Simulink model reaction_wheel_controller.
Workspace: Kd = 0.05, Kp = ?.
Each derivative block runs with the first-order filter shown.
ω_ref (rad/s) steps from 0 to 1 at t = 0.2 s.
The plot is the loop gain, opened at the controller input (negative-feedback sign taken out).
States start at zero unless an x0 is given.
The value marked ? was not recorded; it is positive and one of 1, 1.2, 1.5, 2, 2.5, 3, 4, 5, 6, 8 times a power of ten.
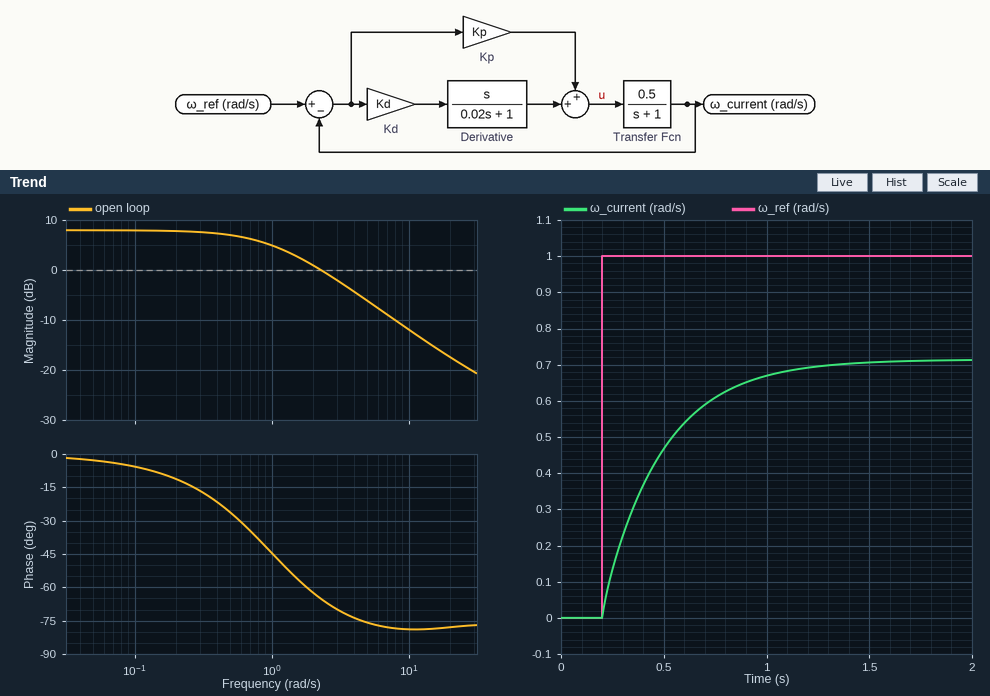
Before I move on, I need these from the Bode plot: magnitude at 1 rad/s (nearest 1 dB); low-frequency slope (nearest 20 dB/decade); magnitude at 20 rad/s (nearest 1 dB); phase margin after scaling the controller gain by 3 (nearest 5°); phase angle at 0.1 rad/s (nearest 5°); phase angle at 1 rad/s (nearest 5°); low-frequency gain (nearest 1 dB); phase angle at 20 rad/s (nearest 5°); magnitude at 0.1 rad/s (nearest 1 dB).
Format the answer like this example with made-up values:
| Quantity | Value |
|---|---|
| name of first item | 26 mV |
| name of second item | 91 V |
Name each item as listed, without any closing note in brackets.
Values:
| Quantity | Value |
|---|---|
| magnitude at 1 rad/s | 5 dB |
| low-frequency slope | 0 dB/decade |
| magnitude at 20 rad/s | -17 dB |
| phase margin after scaling the controller gain by 3 | 100° |
| phase angle at 0.1 rad/s | -5° |
| phase angle at 1 rad/s | -45° |
| low-frequency gain | 8 dB |
| phase angle at 20 rad/s | -80° |
| magnitude at 0.1 rad/s | 8 dB |
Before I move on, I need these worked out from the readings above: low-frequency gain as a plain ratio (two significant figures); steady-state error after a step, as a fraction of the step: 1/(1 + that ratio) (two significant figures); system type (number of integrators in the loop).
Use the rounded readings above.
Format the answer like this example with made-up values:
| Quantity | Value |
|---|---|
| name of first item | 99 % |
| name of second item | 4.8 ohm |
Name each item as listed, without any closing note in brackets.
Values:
| Quantity | Value |
|---|---|
| low-frequency gain as a plain ratio | 2.5 |
| steady-state error after a step, as a fraction of the step: 1/(1 + that ratio) | 0.29 |
| system type | 0 |
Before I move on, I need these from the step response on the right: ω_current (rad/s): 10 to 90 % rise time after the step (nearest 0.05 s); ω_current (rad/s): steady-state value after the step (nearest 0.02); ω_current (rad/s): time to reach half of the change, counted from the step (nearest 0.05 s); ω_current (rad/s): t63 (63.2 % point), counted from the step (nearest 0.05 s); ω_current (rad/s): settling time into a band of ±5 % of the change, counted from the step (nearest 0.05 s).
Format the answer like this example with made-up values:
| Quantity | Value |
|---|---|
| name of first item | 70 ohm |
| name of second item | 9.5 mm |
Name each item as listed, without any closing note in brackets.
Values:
| Quantity | Value |
|---|---|
| ω_current (rad/s): 10 to 90 % rise time after the step | 0.65 s |
| ω_current (rad/s): steady-state value after the step | 0.72 |
| ω_current (rad/s): time to reach half of the change, counted from the step | 0.20 s |
| ω_current (rad/s): t63 (63.2 % point), counted from the step | 0.30 s |
| ω_current (rad/s): settling time into a band of ±5 % of the change, counted from the step | 0.85 s |
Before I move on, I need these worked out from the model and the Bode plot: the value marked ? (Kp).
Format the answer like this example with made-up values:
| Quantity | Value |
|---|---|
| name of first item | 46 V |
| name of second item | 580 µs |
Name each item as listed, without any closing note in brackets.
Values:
| Quantity | Value |
|---|---|
| the value marked ? | 5 |
